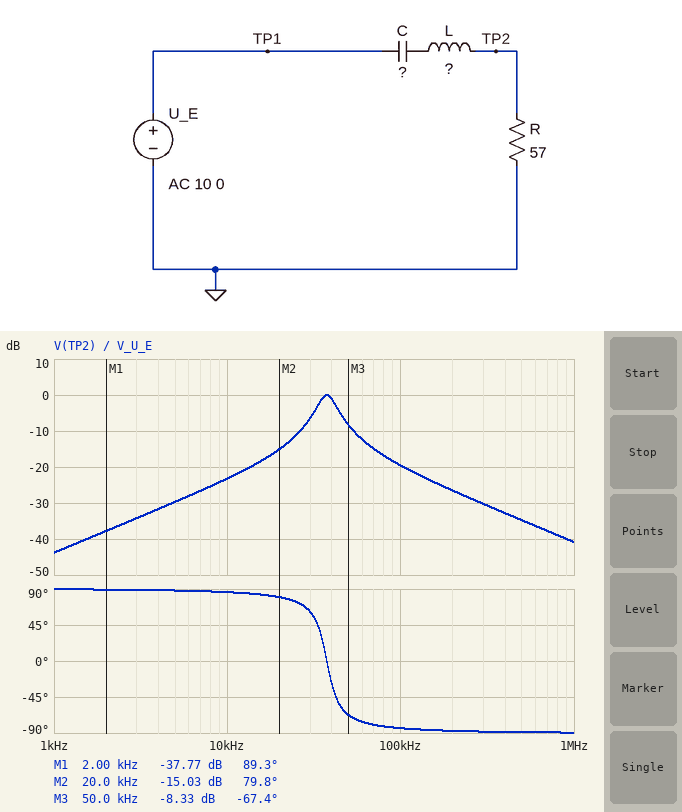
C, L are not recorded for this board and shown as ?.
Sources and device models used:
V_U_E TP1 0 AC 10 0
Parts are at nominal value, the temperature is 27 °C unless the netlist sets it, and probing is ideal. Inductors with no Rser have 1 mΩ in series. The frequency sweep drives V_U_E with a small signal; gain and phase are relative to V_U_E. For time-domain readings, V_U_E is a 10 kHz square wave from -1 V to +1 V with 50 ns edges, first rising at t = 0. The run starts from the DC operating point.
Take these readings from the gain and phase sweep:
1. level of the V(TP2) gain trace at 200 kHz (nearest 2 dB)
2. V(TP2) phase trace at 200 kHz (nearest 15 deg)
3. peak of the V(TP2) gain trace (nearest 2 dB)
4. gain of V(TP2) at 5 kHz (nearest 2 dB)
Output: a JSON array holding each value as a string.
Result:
["-26 dB", "-90 deg", "0 dB", "-30 dB"]
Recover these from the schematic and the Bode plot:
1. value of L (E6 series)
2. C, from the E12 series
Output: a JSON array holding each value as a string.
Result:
["1 mH", "18 nF"]
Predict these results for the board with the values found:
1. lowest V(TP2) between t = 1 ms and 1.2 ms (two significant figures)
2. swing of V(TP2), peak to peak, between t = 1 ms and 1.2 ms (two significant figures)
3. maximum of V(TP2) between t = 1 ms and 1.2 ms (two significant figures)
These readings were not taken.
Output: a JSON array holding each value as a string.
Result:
["-350 mV", "710 mV", "350 mV"]
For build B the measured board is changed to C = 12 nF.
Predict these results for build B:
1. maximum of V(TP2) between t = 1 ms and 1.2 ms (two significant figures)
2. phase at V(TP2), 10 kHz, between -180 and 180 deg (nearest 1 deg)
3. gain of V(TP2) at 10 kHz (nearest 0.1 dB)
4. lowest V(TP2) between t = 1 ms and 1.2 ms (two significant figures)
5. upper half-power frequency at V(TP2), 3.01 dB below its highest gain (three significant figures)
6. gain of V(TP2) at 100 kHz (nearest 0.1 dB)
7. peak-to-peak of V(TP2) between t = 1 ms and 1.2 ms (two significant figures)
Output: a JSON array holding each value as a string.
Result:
["340 mV", "87 deg", "-26.9 dB", "-340 mV", "50.7 kHz", "-18.8 dB", "680 mV"]
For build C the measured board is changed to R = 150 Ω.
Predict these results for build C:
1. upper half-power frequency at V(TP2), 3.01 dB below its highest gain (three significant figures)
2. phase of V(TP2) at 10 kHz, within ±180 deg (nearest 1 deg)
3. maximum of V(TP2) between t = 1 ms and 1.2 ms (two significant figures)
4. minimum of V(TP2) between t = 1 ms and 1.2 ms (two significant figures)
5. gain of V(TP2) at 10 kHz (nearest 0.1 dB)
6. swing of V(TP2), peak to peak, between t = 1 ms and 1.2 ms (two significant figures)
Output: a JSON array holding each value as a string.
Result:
["51.3 kHz", "80 deg", "840 mV", "-840 mV", "-14.9 dB", "1.7 V"]
